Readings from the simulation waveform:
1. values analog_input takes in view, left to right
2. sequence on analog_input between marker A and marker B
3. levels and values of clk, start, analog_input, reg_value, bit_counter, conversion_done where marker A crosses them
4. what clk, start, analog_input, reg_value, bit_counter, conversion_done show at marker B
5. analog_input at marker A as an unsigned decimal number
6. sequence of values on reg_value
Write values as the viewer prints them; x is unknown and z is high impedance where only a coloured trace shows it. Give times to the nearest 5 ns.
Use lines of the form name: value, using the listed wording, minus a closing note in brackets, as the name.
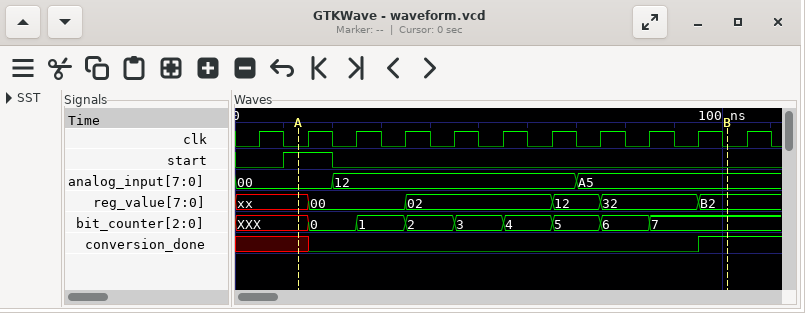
values analog_input takes in view, left to right: 00, 12, A5
sequence on analog_input between marker A and marker B: 00, 12, A5
levels and values of clk, start, analog_input, reg_value, bit_counter, conversion_done where marker A crosses them: clk=0, start=1, analog_input=00, reg_value=xx, bit_counter=XXX, conversion_done=x
what clk, start, analog_input, reg_value, bit_counter, conversion_done show at marker B: clk=0, start=0, analog_input=A5, reg_value=B2, bit_counter=7, conversion_done=1
analog_input at marker A as an unsigned decimal number: 0
sequence of values on reg_value: xx, 00, 02, 12, 32, B2
